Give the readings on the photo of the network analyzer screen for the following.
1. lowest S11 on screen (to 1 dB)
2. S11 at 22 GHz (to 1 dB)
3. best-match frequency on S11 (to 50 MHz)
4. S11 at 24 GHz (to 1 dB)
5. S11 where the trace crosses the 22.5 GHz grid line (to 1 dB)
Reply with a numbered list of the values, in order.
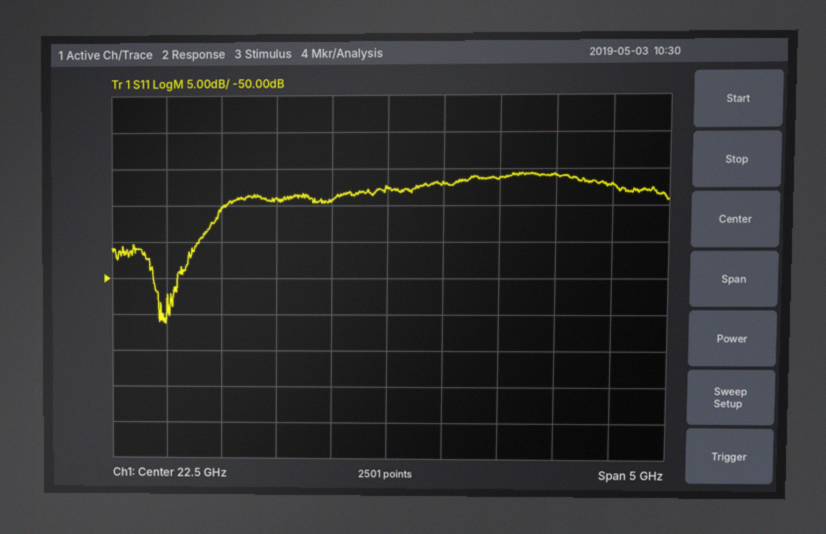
1. -56 dB
2. -39 dB
3. 20.50 GHz
4. -36 dB
5. -38 dB
